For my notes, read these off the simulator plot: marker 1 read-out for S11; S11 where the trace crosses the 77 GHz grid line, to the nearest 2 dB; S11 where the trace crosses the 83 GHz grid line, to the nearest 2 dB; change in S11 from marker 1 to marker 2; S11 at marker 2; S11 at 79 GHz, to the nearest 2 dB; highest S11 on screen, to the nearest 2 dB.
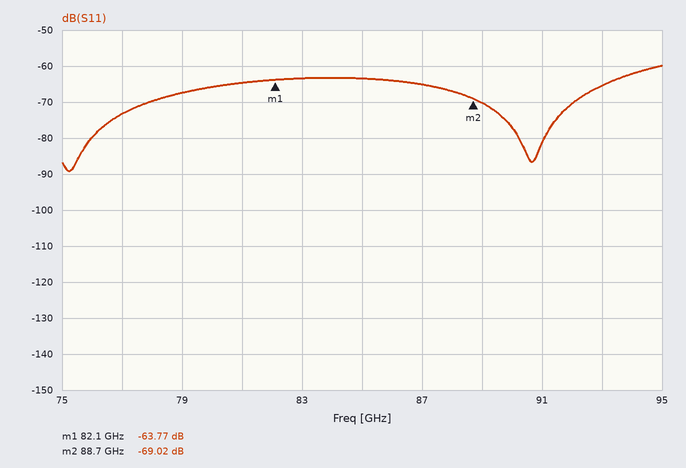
-63.77 dB
-74 dB
-64 dB
-5.25 dB
-69.02 dB
-68 dB
-60 dB
